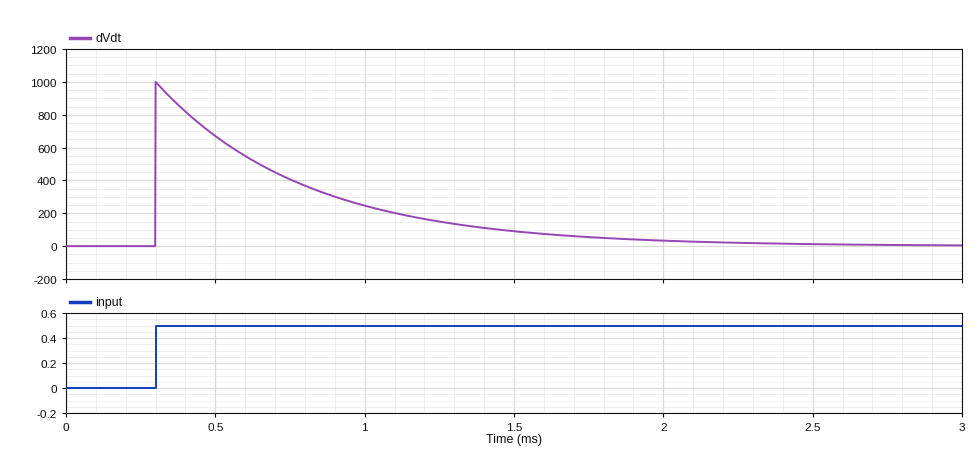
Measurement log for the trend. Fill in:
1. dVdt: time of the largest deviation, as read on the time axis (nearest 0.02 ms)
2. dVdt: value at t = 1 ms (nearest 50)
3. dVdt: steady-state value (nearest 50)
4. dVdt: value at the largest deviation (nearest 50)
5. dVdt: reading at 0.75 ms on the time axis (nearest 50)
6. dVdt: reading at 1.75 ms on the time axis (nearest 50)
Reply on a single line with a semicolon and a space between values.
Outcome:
0.30 ms; 250; 0; 1000; 400; 50
